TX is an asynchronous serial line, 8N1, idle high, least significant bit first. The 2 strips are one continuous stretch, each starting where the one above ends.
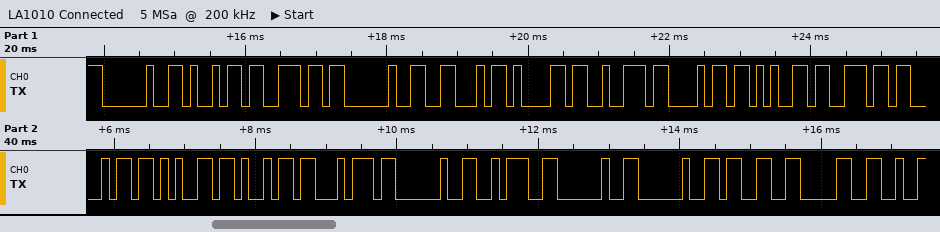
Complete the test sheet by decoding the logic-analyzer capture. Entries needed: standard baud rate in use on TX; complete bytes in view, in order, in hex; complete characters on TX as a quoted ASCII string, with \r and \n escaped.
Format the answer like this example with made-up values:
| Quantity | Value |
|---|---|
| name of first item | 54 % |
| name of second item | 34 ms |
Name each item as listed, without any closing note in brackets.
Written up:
| Quantity | Value |
|---|---|
| standard baud rate in use on TX | 9600 baud |
| complete bytes in view, in order, in hex | 20 69 6E 20 46 61 72 68 65 6E 68 65 69 74 20 3A 20 20 33 30 |
| complete characters on TX as a quoted ASCII string, with \r and \n escaped | " in Farhenheit :  30" |
